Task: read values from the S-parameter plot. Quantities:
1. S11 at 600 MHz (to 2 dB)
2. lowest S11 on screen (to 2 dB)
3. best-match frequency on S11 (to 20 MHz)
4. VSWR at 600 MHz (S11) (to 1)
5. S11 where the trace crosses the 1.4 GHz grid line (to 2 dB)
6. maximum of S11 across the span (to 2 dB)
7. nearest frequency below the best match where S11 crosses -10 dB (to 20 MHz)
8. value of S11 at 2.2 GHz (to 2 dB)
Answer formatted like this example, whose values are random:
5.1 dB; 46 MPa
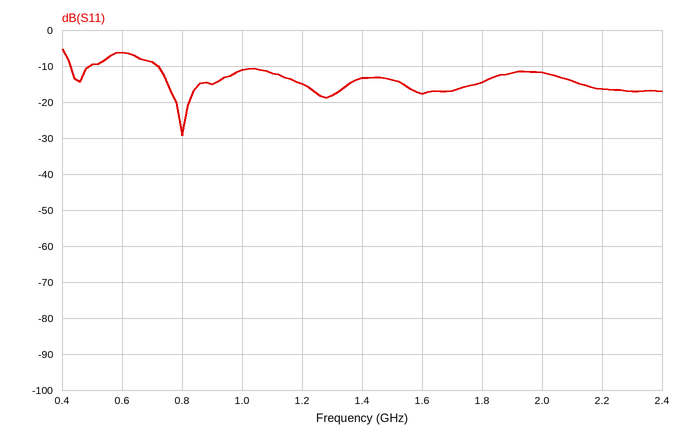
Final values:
-6 dB; -30 dB; 800 MHz; 3; -14 dB; -6 dB; 720 MHz; -16 dB
